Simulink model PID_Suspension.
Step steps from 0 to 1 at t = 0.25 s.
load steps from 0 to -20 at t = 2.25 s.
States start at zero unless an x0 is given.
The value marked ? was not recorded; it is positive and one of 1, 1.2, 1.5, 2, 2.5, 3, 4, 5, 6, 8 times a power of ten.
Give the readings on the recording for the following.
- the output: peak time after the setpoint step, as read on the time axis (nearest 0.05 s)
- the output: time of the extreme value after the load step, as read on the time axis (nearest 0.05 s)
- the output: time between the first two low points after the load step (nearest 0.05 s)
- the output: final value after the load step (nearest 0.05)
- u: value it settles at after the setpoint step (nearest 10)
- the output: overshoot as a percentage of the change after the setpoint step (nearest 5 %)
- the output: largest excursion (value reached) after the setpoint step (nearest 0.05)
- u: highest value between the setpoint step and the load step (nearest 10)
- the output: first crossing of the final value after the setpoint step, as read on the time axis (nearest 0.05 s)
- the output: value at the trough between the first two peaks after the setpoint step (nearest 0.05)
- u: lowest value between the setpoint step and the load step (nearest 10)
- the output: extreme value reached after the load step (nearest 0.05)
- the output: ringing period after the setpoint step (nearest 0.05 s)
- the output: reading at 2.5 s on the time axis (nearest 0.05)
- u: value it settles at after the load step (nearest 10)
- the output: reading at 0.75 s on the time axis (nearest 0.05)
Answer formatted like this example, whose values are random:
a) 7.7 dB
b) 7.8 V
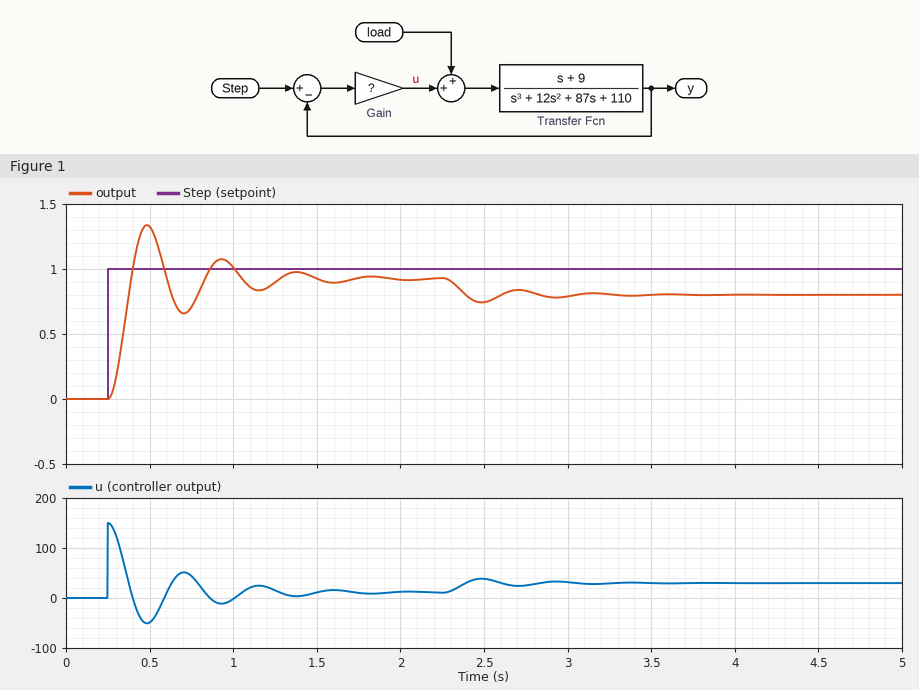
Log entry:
a) 0.50 s
b) 2.50 s
c) 0.45 s
d) 0.80
e) 10
f) 45 %
g) 1.35
h) 150
i) 0.40 s
j) 0.65
k) -50
l) 0.75
m) 0.45 s
n) 0.75
o) 30
p) 0.70
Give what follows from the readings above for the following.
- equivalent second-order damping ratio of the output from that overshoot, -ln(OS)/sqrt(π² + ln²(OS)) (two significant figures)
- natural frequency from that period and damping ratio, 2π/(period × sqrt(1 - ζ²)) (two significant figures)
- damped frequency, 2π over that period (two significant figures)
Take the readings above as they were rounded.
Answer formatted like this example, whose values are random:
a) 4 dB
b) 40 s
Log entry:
a) 0.25
b) 14 rad/s
c) 14 rad/s
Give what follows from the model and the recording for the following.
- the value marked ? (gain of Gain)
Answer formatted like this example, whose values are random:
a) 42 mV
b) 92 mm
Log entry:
a) 150
